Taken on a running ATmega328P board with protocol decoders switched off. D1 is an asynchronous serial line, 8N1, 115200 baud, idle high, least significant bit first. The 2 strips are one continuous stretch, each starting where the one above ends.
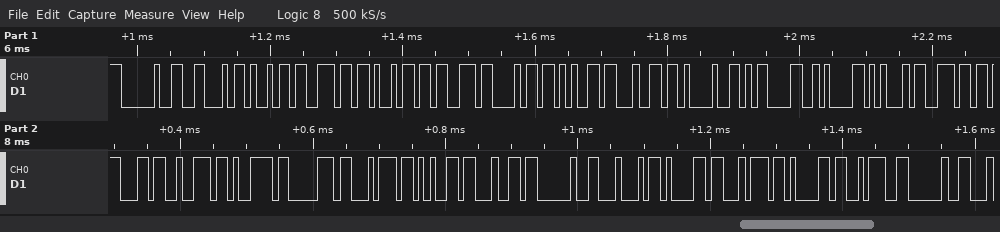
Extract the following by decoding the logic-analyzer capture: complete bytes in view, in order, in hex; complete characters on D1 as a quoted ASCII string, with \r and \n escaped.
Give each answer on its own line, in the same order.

20 46 69 6E 69 73 68 65 64 21 0D 0A 45 6E 63 72 79 70 74 65 64 20 44 61 74 61 3A 20
" Finished!\r\nEncrypted Data: "
